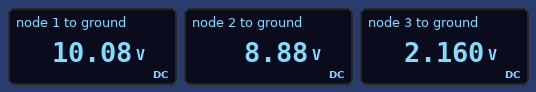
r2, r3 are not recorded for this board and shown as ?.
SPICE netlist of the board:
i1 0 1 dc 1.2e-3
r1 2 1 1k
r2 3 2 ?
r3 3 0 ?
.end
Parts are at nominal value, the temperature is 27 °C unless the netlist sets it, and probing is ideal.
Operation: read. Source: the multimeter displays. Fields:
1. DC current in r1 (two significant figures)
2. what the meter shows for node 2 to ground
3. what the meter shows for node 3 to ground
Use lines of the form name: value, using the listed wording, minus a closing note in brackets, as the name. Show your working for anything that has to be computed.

DC current in r1: (10.08 V - 8.88 V) / 1 kΩ = 1.2 mA
what the meter shows for node 2 to ground: 8.88 V
what the meter shows for node 3 to ground: 2.160 V
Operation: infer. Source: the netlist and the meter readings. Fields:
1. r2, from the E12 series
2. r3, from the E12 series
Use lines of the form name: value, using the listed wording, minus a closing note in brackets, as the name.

r2, from the E12 series: 5.6 kΩ
r3, from the E12 series: 1.8 kΩ
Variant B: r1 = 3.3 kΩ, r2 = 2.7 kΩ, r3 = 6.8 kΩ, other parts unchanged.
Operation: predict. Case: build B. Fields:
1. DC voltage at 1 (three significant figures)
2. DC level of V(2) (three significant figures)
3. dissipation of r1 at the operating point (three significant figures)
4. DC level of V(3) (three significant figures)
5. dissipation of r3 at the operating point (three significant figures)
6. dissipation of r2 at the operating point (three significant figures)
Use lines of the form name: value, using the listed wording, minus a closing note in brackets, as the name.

DC voltage at 1: 15.4 V
DC level of V(2): 11.4 V
dissipation of r1 at the operating point: 4.75 mW
DC level of V(3): 8.16 V
dissipation of r3 at the operating point: 9.79 mW
dissipation of r2 at the operating point: 3.89 mW
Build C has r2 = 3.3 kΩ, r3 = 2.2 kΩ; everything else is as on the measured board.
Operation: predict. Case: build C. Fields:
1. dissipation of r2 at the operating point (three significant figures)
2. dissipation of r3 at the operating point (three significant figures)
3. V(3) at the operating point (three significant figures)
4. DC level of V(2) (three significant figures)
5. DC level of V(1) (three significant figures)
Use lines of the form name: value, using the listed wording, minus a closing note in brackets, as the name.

dissipation of r2 at the operating point: 4.75 mW
dissipation of r3 at the operating point: 3.17 mW
V(3) at the operating point: 2.64 V
DC level of V(2): 6.60 V
DC level of V(1): 7.80 V
